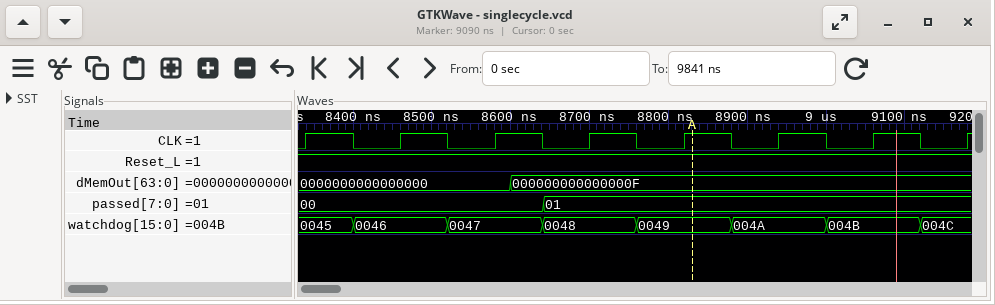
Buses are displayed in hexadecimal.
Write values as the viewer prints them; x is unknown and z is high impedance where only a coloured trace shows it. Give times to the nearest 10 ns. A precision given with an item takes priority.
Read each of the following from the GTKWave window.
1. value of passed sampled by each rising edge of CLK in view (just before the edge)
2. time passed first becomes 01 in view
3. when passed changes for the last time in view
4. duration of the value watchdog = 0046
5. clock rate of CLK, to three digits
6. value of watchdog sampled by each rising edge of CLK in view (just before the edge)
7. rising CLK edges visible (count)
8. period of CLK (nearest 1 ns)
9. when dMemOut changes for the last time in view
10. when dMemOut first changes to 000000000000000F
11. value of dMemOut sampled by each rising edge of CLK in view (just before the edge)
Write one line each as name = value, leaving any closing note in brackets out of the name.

value of passed sampled by each rising edge of CLK in view = 00, 00, 00, 01, 01, 01, 01, 01
time passed first becomes 01 in view = 8640 ns
when passed changes for the last time in view = 8640 ns
duration of the value watchdog = 0046 = 120 ns
clock rate of CLK, to three digits = 8.33 MHz
value of watchdog sampled by each rising edge of CLK in view = 0045, 0046, 0047, 0048, 0049, 004A, 004B, 004C
rising CLK edges visible = 8
period of CLK = 120 ns
when dMemOut changes for the last time in view = 8600 ns
when dMemOut first changes to 000000000000000F = 8600 ns
value of dMemOut sampled by each rising edge of CLK in view = 0000000000000000, 0000000000000000, 0000000000000000, 000000000000000F, 000000000000000F, 000000000000000F, 000000000000000F, 000000000000000F
